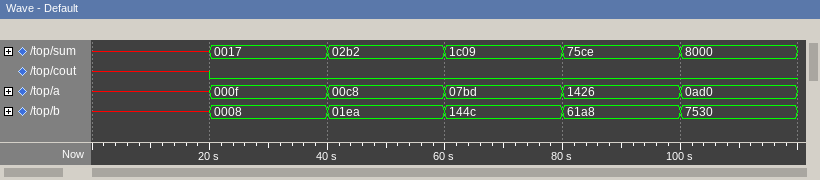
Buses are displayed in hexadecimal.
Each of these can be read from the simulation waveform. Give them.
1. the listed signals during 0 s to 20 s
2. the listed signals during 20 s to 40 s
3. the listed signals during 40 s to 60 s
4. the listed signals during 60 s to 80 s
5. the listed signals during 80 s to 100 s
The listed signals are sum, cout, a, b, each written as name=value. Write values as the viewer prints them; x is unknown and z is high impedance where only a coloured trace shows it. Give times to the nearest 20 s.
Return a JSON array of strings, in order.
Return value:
["sum=x, cout=x, a=x, b=x", "sum=0017, cout=0, a=000f, b=0008", "sum=02b2, cout=0, a=00c8, b=01ea", "sum=1c09, cout=0, a=07bd, b=144c", "sum=75ce, cout=0, a=1426, b=61a8"]
